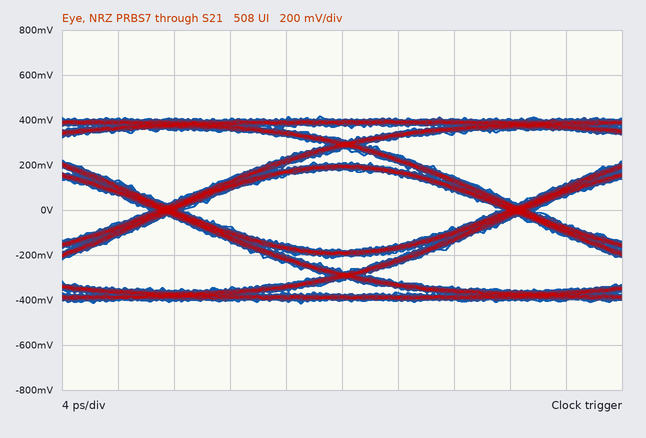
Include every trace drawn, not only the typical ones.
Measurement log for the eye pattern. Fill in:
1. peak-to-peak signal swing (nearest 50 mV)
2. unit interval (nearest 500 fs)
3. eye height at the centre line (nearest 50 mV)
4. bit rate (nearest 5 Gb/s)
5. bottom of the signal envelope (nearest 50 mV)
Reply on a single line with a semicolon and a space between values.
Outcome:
850 mV; 25.0 ps; 350 mV; 40 Gb/s; -400 mV
